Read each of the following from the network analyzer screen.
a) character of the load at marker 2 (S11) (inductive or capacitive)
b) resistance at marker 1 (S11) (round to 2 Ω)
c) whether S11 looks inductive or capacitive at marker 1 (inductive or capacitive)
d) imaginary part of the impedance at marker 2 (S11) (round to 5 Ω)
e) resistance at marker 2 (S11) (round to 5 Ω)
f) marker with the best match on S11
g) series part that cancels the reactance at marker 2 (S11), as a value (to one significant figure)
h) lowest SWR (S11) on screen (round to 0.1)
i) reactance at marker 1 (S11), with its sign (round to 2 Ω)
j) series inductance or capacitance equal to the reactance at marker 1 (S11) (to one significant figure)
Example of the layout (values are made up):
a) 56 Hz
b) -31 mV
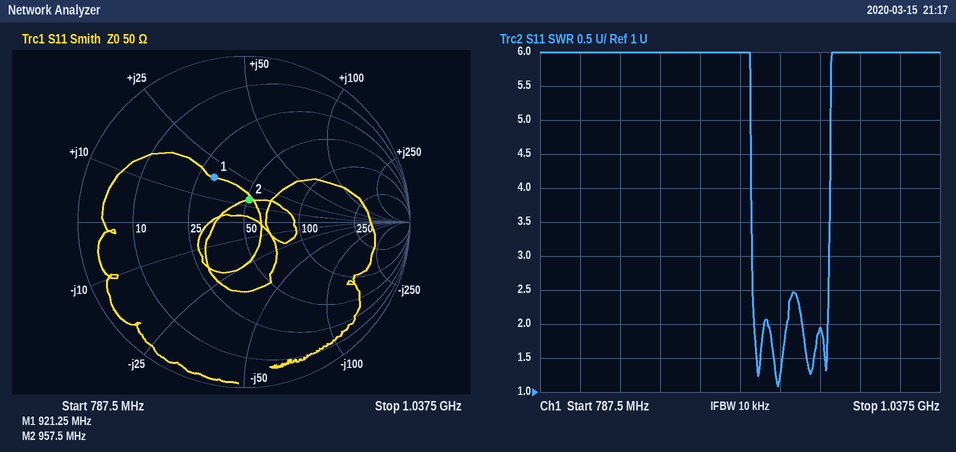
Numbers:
a) inductive
b) 30 Ω
c) inductive
d) +15 Ω
e) 50 Ω
f) marker 2
g) 10 pF
h) 1.1
i) +18 Ω
j) 3 nH
